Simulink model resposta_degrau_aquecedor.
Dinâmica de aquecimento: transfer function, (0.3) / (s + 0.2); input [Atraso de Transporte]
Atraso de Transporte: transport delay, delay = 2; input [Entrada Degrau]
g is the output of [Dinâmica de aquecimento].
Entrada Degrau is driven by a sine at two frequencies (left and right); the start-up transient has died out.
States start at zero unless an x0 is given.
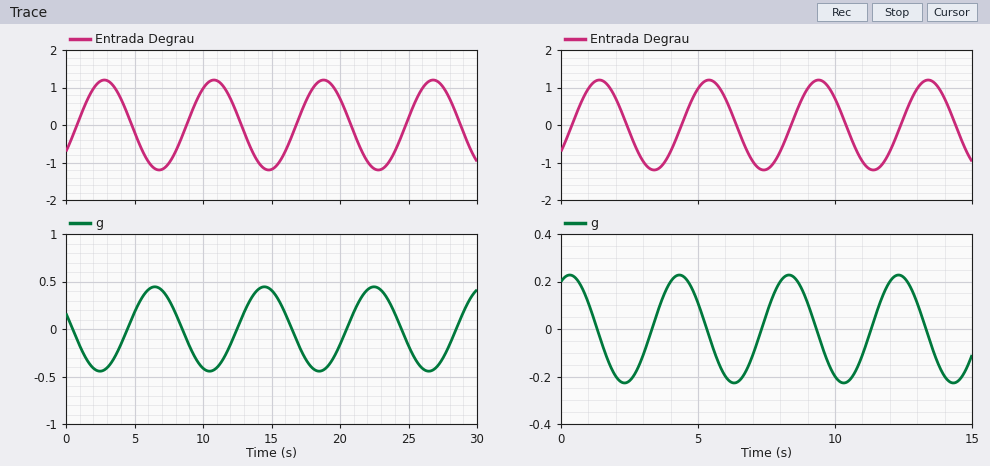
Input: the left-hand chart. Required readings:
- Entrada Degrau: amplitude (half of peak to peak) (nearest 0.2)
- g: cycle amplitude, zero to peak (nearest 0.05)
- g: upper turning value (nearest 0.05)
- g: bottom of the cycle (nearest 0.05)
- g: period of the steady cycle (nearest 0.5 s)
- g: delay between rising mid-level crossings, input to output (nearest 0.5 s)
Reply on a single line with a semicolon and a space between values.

1.2; 0.45; 0.45; -0.45; 8.0 s; 3.5 s
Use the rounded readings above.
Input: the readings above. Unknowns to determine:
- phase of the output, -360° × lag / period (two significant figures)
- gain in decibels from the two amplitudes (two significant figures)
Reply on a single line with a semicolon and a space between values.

-160°; -8.5 dB
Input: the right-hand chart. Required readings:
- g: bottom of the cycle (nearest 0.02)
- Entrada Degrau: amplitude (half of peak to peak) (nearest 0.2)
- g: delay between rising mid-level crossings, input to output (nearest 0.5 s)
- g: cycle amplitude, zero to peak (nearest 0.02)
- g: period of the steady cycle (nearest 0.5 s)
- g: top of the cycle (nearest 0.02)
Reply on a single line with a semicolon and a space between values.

-0.22; 1.2; 3.0 s; 0.22; 4.0 s; 0.22
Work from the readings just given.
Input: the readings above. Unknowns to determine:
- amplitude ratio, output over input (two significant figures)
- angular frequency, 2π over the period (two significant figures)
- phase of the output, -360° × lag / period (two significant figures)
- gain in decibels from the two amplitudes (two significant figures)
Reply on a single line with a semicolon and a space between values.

0.18; 1.6 rad/s; -270°; -15 dB
